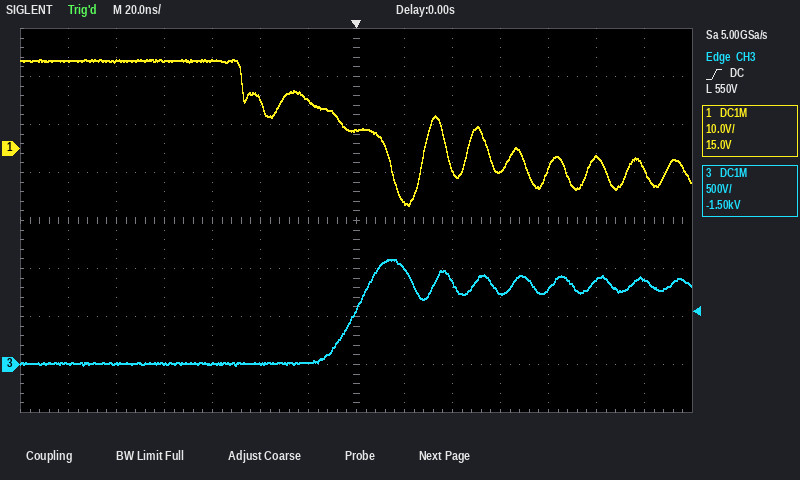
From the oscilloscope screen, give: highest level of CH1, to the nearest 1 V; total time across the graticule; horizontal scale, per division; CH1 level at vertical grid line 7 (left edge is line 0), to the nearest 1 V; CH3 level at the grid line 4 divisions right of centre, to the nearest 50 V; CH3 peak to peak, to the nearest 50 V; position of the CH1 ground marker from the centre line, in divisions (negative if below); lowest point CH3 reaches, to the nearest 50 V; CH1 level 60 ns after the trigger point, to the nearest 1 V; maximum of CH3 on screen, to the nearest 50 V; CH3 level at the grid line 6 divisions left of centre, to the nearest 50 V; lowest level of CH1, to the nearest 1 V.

19 V
280 ns
20 ns
4 V
800 V
1.10 kV
+1.5 div
0 V
-5 V
1.10 kV
0 V
-12 V
